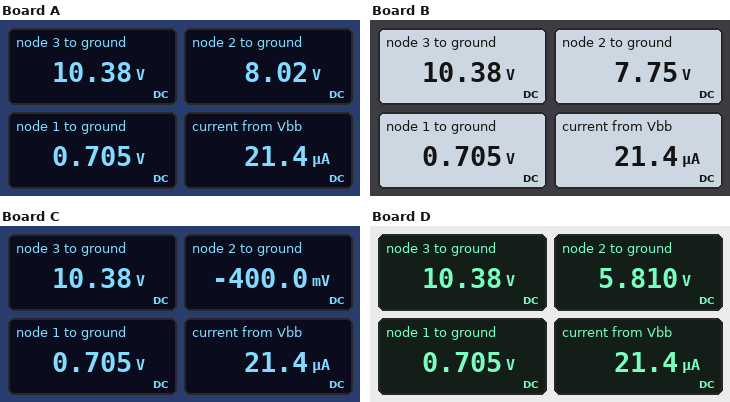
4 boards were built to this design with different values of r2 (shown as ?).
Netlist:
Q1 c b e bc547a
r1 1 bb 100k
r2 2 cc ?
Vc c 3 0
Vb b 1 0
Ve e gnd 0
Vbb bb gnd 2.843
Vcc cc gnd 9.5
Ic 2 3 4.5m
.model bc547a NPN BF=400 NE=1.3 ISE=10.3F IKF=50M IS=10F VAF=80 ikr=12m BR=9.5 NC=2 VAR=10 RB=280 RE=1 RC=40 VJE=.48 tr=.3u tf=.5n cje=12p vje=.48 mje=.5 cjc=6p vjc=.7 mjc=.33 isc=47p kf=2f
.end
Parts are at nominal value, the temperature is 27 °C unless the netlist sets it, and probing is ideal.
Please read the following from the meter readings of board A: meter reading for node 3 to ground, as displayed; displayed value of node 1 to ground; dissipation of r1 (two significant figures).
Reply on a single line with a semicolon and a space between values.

10.38 V; 0.705 V; 46 µW
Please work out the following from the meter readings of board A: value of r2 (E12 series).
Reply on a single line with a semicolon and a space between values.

330 Ω
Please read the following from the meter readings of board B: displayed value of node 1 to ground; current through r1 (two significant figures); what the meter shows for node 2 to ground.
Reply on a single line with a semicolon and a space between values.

0.705 V; 21 µA; 7.75 V
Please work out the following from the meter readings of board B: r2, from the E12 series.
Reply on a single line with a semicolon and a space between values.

390 Ω
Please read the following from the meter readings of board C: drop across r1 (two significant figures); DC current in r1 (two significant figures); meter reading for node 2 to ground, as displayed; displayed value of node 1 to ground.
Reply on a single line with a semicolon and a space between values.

2.1 V; 21 µA; -400.0 mV; 0.705 V
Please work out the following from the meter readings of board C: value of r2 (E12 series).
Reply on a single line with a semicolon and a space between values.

2.2 kΩ
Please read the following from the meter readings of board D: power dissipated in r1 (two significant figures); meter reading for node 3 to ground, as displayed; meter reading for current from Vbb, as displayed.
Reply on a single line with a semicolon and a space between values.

46 µW; 10.38 V; 21.4 µA
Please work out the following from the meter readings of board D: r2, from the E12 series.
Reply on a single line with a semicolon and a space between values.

820 Ω
